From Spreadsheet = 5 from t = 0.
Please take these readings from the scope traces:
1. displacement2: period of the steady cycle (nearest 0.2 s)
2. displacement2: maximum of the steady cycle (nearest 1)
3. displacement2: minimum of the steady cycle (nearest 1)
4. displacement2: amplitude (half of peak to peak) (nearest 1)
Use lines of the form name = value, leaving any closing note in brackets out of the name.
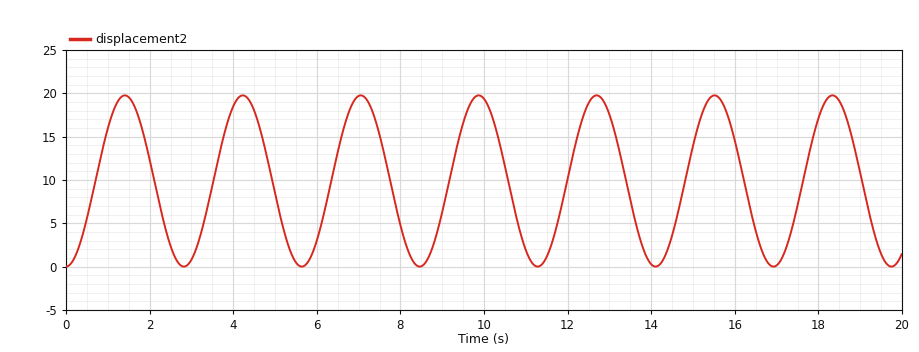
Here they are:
displacement2: period of the steady cycle = 2.8 s
displacement2: maximum of the steady cycle = 20
displacement2: minimum of the steady cycle = 0
displacement2: amplitude (half of peak to peak) = 10
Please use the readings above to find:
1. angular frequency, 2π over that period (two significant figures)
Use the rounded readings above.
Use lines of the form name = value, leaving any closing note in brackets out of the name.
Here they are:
angular frequency, 2π over that period = 2.2 rad/s
